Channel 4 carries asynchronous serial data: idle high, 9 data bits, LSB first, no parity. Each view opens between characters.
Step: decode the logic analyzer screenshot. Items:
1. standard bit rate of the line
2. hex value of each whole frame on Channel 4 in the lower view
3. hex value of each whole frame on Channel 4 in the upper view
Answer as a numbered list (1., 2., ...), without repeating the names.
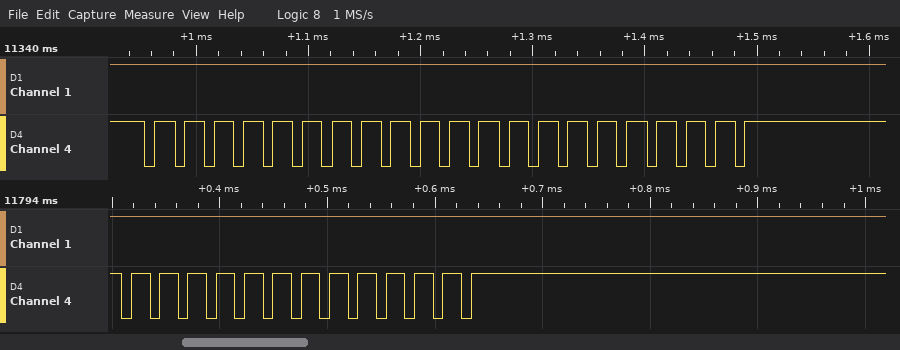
1. 115200 baud
2. DB, DB, DB, 1FF
3. DB, DB, DB, DB, DB, 1FF
